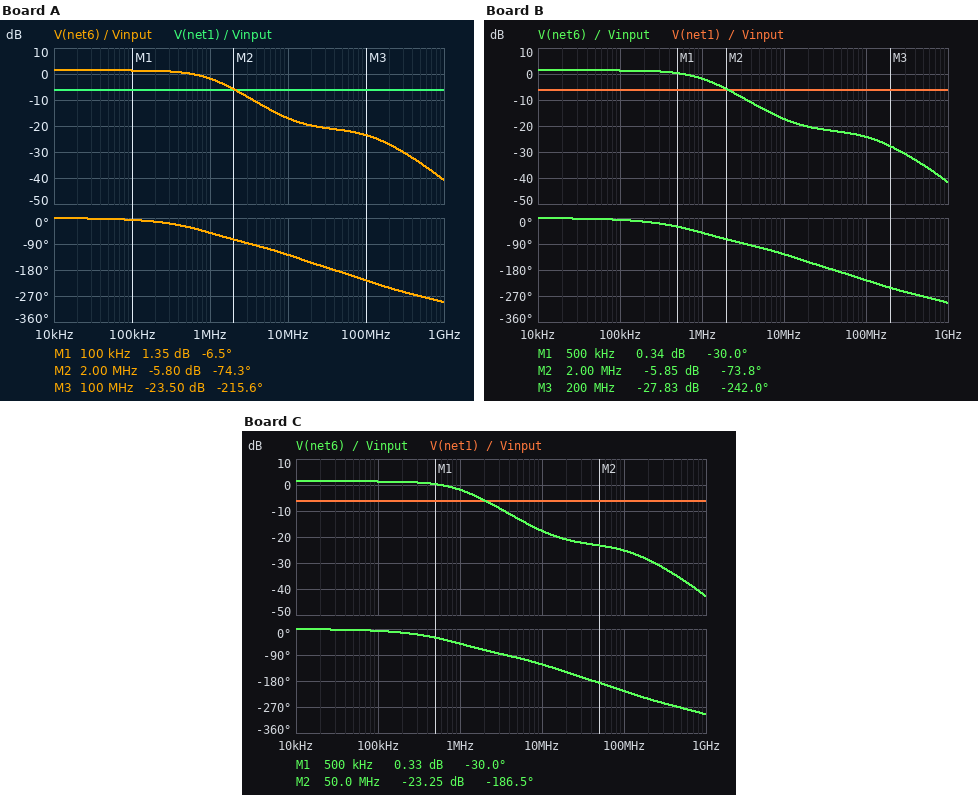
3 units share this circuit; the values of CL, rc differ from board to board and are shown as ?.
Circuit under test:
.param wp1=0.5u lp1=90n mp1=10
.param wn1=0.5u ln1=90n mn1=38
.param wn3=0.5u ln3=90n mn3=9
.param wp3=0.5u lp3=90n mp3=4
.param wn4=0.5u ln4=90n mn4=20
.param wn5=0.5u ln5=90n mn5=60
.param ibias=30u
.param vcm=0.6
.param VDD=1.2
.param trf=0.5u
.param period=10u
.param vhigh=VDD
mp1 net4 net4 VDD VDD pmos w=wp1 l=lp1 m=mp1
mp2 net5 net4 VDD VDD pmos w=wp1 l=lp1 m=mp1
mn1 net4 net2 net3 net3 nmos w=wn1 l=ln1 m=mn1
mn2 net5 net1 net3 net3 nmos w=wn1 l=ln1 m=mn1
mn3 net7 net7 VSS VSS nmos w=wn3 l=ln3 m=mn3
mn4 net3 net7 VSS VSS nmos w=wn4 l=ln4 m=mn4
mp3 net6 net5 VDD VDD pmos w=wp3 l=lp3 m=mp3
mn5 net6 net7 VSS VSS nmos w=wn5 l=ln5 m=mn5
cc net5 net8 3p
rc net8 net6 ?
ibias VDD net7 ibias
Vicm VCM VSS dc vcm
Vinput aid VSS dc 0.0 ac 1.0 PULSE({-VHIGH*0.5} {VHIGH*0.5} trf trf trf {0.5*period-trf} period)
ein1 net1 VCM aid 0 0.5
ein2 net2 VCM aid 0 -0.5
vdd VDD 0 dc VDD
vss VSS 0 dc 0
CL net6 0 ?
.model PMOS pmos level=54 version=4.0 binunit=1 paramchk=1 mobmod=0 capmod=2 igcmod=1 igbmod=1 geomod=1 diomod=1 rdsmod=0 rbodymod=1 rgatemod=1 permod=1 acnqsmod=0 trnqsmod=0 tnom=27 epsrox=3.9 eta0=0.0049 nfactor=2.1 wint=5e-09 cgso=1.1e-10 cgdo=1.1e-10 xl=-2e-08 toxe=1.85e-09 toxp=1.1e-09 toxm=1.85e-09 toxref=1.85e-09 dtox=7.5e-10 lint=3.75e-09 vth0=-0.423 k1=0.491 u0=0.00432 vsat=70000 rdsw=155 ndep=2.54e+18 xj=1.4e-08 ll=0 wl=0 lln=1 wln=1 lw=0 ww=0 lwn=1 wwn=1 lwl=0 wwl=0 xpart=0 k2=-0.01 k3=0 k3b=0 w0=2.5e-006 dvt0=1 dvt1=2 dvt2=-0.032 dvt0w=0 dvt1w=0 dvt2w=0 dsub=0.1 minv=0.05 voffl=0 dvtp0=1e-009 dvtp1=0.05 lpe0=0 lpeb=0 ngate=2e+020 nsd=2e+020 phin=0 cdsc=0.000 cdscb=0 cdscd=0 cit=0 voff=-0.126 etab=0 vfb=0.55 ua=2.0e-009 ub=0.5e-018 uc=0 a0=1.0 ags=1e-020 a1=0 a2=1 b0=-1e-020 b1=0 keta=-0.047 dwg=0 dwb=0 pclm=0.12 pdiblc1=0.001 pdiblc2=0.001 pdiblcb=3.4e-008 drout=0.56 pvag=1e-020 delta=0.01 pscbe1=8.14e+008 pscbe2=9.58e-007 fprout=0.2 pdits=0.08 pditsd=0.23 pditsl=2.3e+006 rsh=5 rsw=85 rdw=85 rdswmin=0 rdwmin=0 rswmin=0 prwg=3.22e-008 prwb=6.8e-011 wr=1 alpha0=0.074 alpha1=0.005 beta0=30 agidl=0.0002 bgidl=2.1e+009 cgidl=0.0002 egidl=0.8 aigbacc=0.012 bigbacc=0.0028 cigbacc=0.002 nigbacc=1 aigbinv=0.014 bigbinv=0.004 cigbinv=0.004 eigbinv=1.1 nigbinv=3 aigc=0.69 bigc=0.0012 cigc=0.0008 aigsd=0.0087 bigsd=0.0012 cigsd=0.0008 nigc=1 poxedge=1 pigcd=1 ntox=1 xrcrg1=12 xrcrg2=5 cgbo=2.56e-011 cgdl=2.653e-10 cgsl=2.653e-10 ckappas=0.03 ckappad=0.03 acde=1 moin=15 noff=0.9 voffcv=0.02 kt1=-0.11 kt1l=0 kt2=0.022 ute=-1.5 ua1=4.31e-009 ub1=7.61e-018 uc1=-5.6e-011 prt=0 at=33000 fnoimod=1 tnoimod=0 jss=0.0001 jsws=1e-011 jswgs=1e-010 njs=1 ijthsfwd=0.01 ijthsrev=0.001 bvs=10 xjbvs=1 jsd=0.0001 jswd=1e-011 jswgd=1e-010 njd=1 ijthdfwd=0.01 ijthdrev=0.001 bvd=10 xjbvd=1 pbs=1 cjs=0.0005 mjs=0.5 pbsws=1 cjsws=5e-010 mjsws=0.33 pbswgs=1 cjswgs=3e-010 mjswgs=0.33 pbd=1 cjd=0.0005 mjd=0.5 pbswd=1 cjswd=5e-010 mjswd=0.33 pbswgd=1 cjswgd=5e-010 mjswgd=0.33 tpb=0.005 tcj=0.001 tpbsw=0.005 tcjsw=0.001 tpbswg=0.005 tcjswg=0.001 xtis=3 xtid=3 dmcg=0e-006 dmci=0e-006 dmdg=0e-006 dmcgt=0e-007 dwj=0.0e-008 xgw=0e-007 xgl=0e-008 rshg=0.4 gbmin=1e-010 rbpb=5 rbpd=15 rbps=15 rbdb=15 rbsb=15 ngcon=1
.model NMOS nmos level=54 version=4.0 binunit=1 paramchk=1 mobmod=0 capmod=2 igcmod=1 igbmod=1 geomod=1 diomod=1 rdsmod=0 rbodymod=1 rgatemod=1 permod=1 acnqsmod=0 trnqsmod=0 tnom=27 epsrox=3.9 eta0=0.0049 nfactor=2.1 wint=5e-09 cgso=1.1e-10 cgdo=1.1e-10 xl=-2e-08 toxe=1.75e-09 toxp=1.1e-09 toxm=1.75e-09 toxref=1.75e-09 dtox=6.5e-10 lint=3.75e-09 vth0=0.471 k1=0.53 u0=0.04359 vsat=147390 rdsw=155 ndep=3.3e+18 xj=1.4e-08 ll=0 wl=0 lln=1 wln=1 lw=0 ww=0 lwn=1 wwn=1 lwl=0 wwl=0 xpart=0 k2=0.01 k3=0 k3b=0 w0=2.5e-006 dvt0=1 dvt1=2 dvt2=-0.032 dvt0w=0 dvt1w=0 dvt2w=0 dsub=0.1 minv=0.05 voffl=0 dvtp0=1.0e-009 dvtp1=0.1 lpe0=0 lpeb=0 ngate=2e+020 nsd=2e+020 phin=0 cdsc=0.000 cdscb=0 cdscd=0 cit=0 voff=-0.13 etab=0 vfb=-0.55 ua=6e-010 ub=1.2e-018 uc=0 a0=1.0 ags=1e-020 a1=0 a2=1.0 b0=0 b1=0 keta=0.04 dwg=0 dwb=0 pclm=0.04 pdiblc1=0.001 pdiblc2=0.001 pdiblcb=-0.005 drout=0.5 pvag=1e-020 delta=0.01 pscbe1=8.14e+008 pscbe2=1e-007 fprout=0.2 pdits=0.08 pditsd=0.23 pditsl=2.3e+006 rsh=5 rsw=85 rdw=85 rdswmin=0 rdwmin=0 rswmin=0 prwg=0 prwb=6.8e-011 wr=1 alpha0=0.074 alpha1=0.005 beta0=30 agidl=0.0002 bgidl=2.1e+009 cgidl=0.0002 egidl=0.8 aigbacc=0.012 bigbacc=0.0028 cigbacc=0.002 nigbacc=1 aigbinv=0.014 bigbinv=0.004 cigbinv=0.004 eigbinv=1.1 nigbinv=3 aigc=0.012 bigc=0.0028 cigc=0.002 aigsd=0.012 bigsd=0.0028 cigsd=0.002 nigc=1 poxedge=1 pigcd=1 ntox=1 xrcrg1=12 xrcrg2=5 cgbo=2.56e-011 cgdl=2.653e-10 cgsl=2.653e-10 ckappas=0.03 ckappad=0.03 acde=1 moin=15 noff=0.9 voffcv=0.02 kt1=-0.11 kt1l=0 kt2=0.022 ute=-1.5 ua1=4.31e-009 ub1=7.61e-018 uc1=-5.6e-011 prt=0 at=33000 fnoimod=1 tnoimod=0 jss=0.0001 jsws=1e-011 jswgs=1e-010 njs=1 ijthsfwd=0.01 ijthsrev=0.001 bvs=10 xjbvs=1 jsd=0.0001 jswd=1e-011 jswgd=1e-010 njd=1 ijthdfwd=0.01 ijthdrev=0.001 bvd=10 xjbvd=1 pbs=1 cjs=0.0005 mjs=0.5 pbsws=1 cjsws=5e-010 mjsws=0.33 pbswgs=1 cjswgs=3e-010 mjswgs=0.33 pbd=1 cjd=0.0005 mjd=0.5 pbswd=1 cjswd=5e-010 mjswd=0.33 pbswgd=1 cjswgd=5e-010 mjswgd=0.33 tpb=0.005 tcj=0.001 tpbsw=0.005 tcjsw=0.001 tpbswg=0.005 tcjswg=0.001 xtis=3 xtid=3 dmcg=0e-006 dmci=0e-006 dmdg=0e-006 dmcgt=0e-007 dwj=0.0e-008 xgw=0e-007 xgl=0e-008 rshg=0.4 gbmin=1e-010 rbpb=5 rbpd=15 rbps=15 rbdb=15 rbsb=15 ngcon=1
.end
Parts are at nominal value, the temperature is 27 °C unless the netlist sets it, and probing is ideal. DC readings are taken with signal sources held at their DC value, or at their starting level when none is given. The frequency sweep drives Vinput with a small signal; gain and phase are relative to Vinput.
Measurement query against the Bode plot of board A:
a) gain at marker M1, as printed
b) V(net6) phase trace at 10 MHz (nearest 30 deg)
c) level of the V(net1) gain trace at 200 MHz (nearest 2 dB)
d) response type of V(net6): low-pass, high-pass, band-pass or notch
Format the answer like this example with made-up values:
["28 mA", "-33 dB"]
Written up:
["1.35 dB", "-120 deg", "-6 dB", "low-pass"]
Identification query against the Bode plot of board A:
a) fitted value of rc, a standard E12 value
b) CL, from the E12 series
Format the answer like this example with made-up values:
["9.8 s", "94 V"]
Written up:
["1.5 kΩ", "6.8 pF"]
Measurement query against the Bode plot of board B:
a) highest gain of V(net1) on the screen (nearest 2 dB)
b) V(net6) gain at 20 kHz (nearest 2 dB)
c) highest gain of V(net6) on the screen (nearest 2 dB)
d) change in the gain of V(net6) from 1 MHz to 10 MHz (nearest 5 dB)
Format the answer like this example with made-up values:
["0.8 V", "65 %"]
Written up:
["-6 dB", "2 dB", "2 dB", "-15 dB"]
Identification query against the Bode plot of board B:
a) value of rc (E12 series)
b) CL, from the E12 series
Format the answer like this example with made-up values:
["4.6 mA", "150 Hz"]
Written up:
["1.8 kΩ", "6.8 pF"]
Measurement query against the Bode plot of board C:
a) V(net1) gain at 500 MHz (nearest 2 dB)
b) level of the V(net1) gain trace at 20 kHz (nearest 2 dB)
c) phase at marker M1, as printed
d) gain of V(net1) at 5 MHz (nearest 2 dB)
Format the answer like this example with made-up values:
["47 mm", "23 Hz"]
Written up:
["-6 dB", "-6 dB", "-30.0 deg", "-6 dB"]
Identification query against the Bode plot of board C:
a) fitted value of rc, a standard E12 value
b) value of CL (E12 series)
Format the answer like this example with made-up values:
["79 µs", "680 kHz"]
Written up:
["2.2 kΩ", "6.8 pF"]
